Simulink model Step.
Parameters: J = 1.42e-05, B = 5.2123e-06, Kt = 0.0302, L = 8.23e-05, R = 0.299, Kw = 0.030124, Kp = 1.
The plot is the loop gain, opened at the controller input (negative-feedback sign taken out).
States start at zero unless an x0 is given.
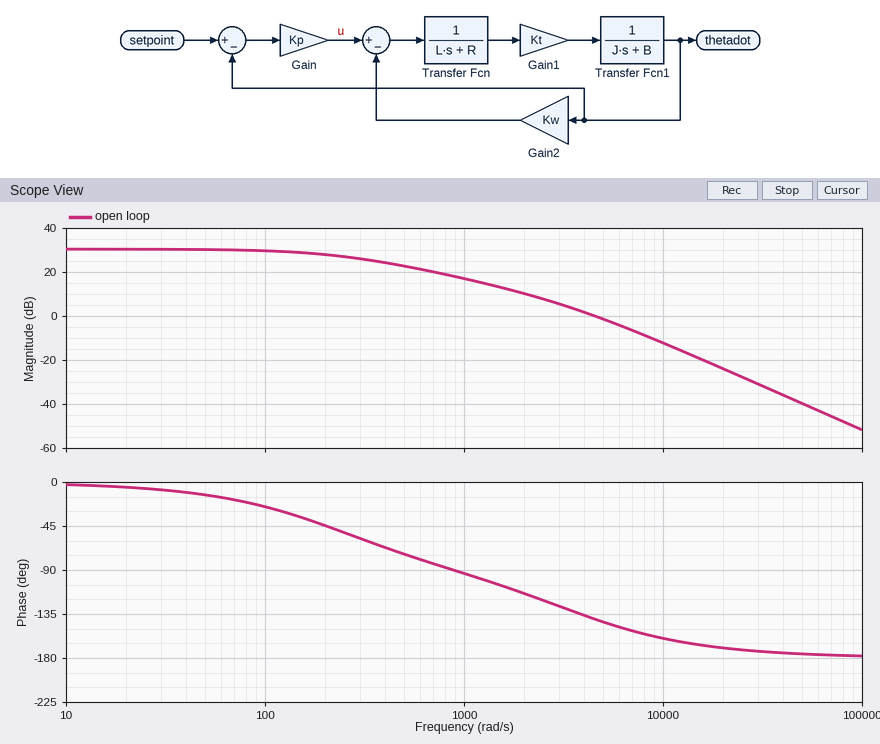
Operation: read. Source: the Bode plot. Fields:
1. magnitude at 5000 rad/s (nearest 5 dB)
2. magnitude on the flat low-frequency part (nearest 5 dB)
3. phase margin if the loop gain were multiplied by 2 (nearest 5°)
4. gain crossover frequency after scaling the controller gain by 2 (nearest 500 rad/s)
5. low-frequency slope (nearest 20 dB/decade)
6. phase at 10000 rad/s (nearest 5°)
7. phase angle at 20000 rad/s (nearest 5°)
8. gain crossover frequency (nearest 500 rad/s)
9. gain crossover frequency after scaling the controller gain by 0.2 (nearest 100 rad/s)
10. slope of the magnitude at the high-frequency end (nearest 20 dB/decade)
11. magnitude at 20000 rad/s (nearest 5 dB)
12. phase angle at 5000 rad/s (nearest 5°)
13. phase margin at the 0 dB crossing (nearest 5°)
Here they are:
0 dB
30 dB
30°
7000 rad/s
0 dB/decade
-160°
-170°
4500 rad/s
1400 rad/s
-40 dB/decade
-25 dB
-145°
40°
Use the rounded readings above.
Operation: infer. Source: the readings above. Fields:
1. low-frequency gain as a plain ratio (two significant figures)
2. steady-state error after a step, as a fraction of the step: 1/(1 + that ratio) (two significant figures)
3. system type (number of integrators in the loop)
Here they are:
32
0.030
0
